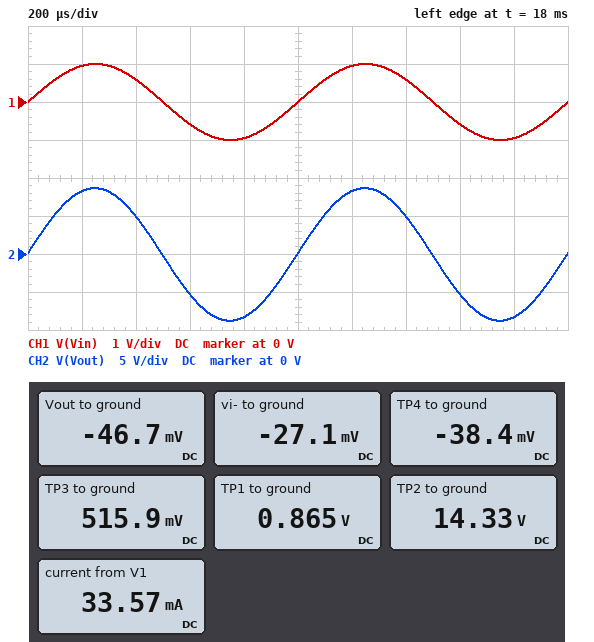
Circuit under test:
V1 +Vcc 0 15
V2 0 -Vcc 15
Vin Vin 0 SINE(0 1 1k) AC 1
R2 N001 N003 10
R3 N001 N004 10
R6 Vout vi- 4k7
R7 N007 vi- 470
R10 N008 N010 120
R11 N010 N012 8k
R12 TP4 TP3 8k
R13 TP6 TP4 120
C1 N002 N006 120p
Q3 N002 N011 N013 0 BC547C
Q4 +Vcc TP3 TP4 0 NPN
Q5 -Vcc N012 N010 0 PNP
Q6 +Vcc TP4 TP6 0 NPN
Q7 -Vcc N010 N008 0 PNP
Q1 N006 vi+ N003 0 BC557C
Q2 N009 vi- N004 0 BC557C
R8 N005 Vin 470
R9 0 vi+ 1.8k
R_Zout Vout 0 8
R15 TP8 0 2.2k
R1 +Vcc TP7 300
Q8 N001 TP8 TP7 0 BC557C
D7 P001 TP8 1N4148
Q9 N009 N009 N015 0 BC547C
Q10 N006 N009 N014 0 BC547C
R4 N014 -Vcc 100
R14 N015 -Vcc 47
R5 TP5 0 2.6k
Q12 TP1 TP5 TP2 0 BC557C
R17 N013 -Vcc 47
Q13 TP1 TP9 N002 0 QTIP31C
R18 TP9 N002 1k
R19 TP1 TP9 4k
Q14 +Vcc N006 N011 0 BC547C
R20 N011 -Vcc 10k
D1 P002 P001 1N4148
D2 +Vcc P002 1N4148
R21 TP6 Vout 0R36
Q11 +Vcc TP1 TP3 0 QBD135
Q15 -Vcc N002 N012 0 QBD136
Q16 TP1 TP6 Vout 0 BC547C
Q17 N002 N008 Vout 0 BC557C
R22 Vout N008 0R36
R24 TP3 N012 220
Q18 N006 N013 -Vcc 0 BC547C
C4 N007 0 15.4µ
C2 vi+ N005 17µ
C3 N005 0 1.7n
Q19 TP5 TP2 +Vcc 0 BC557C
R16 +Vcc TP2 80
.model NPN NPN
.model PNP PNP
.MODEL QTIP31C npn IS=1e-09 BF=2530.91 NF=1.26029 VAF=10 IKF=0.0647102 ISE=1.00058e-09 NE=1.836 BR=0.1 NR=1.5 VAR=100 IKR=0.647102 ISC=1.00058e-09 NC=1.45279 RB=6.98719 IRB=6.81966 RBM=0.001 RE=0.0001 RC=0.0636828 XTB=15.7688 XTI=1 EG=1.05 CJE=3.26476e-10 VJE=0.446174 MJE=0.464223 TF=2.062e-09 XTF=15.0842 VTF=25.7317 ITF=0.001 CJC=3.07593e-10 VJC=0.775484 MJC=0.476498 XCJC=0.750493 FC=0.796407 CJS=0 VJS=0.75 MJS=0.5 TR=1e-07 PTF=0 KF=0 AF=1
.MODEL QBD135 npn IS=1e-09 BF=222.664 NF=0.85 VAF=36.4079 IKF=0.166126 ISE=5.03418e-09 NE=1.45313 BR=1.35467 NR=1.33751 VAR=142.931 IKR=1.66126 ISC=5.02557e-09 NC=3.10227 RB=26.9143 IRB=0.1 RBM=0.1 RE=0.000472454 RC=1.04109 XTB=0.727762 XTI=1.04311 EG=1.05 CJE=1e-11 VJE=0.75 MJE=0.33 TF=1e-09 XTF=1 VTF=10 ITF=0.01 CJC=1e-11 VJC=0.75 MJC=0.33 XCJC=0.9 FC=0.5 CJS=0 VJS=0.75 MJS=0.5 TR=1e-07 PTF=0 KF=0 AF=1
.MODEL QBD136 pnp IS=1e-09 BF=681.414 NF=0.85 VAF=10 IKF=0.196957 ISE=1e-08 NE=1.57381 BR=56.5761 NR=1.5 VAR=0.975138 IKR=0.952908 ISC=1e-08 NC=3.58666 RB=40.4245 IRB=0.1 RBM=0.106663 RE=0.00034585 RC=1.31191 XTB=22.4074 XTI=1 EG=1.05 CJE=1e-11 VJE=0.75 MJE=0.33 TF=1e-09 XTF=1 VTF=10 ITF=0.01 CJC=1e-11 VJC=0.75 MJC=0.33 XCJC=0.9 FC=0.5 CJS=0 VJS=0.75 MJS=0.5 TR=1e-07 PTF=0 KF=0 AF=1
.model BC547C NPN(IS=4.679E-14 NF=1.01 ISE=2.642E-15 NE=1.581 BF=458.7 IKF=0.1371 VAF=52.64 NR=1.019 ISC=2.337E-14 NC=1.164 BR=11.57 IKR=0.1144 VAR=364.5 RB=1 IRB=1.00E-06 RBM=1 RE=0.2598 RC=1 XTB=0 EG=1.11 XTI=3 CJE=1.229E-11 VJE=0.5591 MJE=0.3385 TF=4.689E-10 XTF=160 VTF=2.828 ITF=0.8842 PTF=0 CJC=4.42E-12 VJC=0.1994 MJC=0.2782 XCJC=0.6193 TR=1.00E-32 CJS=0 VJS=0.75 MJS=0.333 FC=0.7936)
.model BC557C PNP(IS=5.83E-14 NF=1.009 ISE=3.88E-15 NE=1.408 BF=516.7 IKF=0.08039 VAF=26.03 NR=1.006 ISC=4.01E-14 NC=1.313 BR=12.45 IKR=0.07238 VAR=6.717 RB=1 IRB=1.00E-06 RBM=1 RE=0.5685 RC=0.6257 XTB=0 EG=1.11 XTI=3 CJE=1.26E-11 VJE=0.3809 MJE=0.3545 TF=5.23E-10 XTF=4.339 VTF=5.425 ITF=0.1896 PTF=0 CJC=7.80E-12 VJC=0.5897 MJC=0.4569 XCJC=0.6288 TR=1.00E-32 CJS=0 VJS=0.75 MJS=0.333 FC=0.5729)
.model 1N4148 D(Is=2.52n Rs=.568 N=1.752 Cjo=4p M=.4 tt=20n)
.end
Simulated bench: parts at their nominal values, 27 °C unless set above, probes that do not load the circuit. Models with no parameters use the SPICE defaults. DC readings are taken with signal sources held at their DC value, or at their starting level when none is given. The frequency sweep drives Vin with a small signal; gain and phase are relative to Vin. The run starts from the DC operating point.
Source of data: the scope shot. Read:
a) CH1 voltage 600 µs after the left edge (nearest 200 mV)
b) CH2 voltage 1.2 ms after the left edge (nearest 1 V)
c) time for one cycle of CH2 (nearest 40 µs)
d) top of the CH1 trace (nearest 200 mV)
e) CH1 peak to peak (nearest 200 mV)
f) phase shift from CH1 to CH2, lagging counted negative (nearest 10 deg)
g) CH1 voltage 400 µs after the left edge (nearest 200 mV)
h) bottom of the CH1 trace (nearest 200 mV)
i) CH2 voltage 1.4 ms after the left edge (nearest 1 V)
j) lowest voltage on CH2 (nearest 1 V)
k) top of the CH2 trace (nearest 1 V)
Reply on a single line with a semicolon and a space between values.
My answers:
-600 mV; 8 V; 1.00 ms; 1.0 V; 2.0 V; 0 deg; 600 mV; -1.0 V; 5 V; -9 V; 9 V
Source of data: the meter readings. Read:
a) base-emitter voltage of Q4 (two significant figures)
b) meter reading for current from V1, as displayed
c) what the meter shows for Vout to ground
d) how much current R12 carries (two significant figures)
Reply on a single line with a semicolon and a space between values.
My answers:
550 mV; 33.57 mA; -46.7 mV; 69 µA
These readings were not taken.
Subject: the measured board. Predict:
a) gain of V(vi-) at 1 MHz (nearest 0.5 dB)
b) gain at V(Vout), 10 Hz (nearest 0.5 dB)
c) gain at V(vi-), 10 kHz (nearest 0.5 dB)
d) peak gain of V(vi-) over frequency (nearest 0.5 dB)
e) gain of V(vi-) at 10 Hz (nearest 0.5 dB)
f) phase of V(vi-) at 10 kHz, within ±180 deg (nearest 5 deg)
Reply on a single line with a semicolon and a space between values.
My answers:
-27.0 dB; 10.5 dB; -2.0 dB; -2.0 dB; -2.5 dB; -5 deg
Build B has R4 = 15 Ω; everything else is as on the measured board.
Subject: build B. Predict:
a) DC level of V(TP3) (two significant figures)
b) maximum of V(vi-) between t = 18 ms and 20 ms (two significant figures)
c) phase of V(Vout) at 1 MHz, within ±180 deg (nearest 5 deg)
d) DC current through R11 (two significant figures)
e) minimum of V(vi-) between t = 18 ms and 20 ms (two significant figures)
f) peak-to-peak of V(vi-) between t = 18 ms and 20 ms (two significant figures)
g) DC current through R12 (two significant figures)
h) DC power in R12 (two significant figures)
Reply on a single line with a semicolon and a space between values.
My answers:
1.4 V; 840 mV; -140 deg; 86 µA; -750 mV; 1.6 V; 100 µA; 83 µW
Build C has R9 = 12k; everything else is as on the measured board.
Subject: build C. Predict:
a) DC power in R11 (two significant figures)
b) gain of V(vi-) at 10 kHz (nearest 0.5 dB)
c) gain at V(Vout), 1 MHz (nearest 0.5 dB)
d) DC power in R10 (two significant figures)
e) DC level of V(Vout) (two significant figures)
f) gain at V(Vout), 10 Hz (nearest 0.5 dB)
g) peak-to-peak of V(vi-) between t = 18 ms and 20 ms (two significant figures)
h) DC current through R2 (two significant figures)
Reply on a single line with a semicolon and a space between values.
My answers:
81 µW; -0.5 dB; -2.5 dB; 1.6 mW; -24 mV; 13.0 dB; 1.9 V; 1.6 mA
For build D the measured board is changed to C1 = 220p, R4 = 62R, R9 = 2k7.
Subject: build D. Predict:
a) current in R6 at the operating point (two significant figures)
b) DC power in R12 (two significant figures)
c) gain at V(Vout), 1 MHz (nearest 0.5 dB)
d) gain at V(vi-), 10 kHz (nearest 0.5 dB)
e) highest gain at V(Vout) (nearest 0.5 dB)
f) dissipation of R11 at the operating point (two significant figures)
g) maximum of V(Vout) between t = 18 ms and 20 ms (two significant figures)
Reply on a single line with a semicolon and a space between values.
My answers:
3.5 µA; 74 µW; -5.0 dB; -1.5 dB; 19.5 dB; 81 µW; 9.3 V
